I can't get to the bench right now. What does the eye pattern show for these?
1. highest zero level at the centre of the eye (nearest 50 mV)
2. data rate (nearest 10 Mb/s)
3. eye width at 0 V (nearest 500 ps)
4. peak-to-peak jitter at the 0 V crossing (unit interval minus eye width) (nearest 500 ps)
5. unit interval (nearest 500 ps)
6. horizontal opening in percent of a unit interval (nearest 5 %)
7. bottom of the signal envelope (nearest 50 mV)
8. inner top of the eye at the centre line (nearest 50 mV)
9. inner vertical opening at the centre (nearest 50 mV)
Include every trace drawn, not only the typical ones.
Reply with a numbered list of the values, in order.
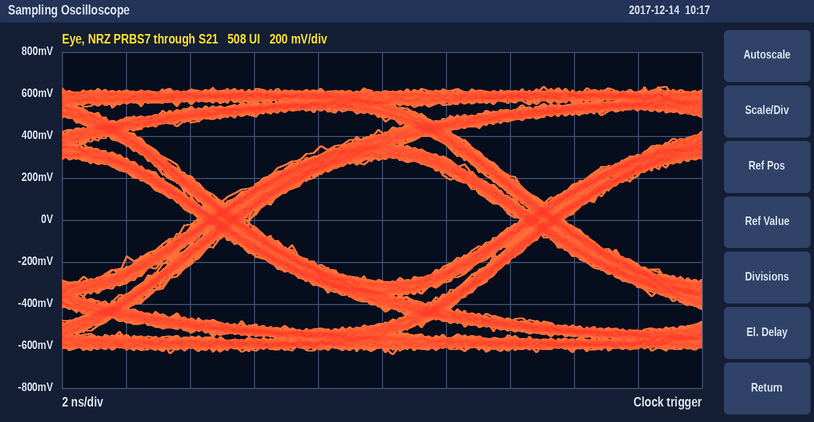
1. -300 mV
2. 100 Mb/s
3. 8.5 ns
4. 1.5 ns
5. 10.0 ns
6. 85 %
7. -650 mV
8. 300 mV
9. 600 mV
